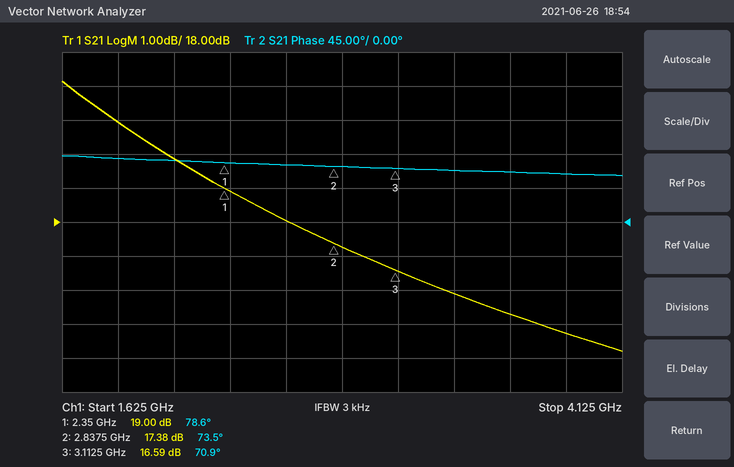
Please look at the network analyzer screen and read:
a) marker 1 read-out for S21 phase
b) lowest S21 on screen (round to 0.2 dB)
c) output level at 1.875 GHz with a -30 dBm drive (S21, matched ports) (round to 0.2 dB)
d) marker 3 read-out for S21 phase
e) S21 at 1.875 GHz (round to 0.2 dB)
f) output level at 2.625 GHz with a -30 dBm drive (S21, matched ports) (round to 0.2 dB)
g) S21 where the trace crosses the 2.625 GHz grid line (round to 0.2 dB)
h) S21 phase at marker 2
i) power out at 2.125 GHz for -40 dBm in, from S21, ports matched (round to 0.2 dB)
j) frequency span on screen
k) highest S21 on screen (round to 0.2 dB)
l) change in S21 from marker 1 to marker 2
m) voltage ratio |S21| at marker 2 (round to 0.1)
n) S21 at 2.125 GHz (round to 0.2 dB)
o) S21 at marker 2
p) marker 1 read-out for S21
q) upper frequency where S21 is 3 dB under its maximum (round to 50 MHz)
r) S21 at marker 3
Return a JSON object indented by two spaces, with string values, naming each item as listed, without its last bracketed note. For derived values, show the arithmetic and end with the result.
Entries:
{
  "marker 1 read-out for S21 phase": "78.6°",
  "lowest S21 on screen": "14.2 dB",
  "output level at 1.875 GHz with a -30 dBm drive (S21, matched ports)": "-30 dBm + (21.0 dB) = -9.0 dBm",
  "marker 3 read-out for S21 phase": "70.9°",
  "S21 at 1.875 GHz": "21.0 dB",
  "output level at 2.625 GHz with a -30 dBm drive (S21, matched ports)": "-30 dBm + (18.0 dB) = -12.0 dBm",
  "S21 where the trace crosses the 2.625 GHz grid line": "18.0 dB",
  "S21 phase at marker 2": "73.5°",
  "power out at 2.125 GHz for -40 dBm in, from S21, ports matched": "-40 dBm + (19.8 dB) = -20.2 dBm",
  "frequency span on screen": "2.5 GHz",
  "highest S21 on screen": "22.2 dB",
  "change in S21 from marker 1 to marker 2": "17.38 − (19) = -1.62 dB",
  "voltage ratio |S21| at marker 2": "10^(17.38/20) ≈ 7.4",
  "S21 at 2.125 GHz": "19.8 dB",
  "S21 at marker 2": "17.38 dB",
  "marker 1 read-out for S21": "19.00 dB",
  "upper frequency where S21 is 3 dB under its maximum": "2.30 GHz",
  "S21 at marker 3": "16.59 dB"
}
